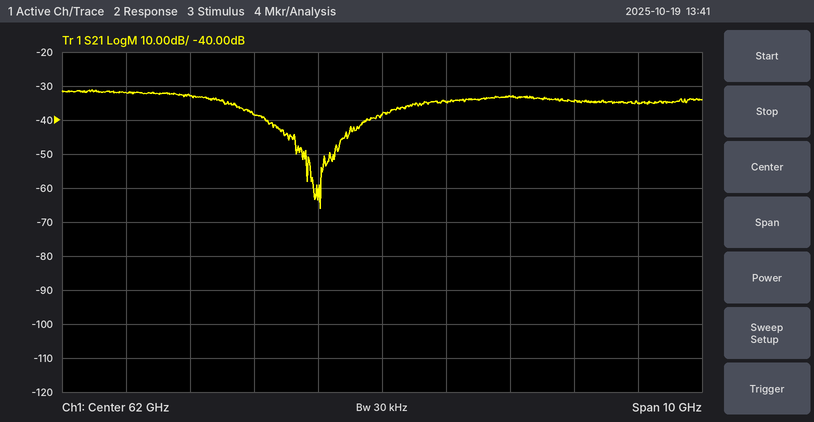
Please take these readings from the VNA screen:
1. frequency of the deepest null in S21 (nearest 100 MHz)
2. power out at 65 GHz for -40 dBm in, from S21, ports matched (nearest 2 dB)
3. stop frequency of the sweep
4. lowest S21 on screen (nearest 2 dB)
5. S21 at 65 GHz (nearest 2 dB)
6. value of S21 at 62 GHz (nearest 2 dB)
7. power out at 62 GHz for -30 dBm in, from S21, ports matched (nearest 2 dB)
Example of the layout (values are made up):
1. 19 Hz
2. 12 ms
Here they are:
1. 61.0 GHz
2. -74 dBm
3. 67 GHz
4. -66 dB
5. -34 dB
6. -38 dB
7. -68 dBm
